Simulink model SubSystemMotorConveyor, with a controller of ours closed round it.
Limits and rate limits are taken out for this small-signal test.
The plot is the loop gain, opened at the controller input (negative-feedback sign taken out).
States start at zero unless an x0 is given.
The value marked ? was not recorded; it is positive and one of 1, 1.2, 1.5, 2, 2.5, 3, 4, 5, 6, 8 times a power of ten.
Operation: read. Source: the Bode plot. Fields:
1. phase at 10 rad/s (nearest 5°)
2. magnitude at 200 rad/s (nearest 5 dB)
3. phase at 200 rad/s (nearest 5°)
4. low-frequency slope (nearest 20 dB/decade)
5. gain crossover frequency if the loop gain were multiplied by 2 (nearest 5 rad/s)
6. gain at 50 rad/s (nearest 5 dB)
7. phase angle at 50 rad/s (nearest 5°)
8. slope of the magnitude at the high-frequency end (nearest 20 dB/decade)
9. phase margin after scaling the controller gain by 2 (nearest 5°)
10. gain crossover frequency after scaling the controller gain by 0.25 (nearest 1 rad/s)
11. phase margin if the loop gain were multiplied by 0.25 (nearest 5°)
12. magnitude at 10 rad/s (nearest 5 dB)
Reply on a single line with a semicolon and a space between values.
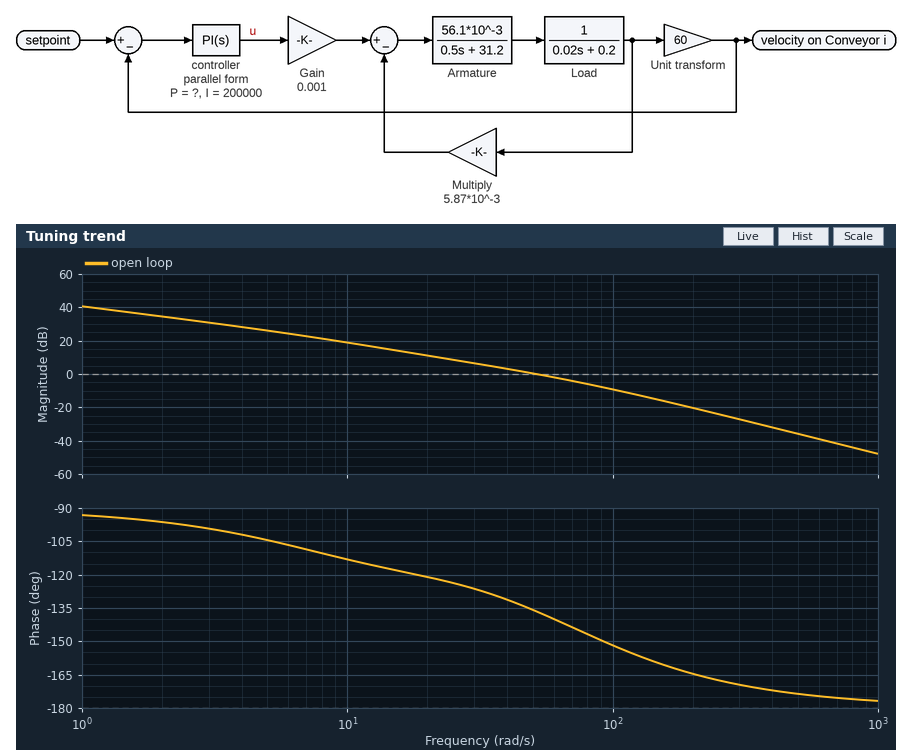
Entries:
-115°; -20 dB; -165°; -20 dB/decade; 80 rad/s; 0 dB; -135°; -40 dB/decade; 35°; 18 rad/s; 60°; 20 dB
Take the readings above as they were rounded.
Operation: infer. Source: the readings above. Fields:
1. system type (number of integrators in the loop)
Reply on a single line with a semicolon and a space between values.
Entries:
1
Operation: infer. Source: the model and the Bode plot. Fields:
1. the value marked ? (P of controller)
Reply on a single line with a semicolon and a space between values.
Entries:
12000
